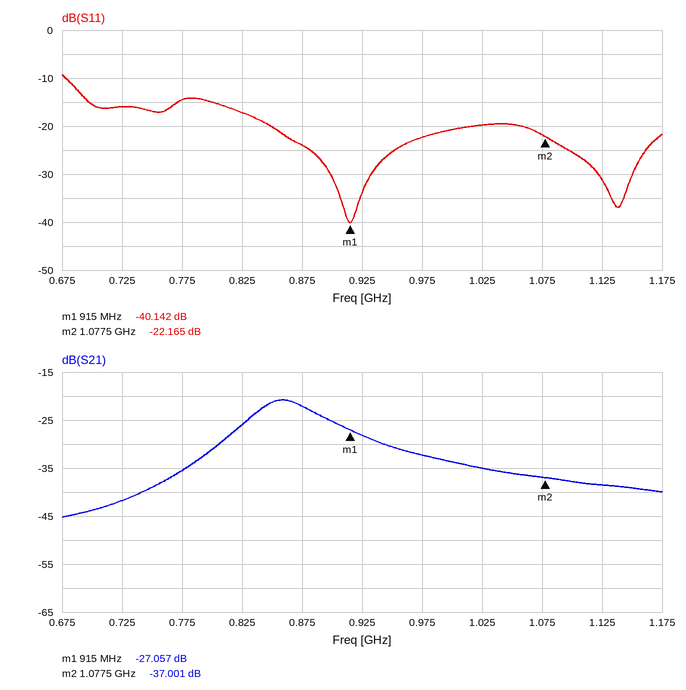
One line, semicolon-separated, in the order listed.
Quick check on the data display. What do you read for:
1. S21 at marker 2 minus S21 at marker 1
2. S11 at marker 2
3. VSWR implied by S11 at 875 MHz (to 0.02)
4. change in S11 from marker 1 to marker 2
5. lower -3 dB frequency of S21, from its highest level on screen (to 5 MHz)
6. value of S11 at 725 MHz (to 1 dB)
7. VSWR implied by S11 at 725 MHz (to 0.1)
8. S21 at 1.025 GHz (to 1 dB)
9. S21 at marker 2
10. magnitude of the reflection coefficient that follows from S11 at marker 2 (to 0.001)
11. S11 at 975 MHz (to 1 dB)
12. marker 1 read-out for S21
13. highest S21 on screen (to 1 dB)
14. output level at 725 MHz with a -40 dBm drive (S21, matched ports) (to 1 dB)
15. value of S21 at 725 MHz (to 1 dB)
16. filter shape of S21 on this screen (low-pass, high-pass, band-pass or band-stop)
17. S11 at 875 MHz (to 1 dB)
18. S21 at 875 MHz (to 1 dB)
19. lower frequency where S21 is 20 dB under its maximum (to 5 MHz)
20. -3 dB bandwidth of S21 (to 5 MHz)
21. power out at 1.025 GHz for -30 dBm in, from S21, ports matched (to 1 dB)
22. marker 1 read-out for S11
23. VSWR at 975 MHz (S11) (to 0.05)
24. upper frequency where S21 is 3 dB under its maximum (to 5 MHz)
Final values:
-9.944 dB; -22.165 dB; 1.14; 17.977 dB; 835 MHz; -16 dB; 1.4; -35 dB; -37.001 dB; 0.078; -22 dB; -27.057 dB; -21 dB; -82 dBm; -42 dB; band-pass; -24 dB; -22 dB; 735 MHz; 55 MHz; -65 dBm; -40.142 dB; 1.15; 890 MHz
